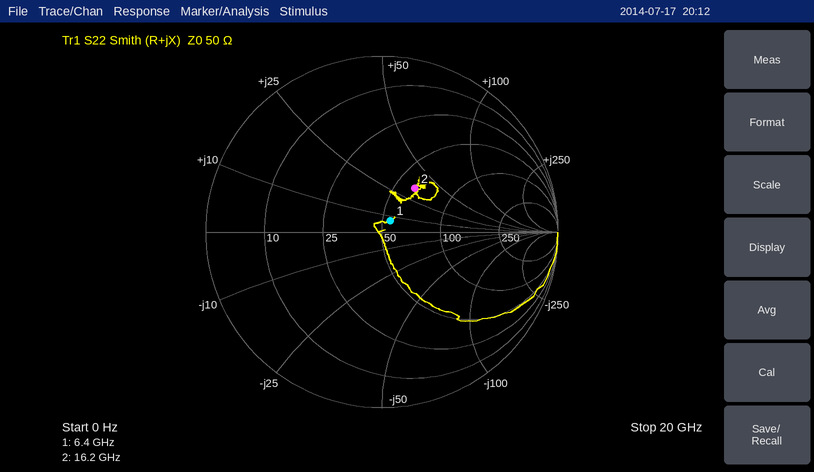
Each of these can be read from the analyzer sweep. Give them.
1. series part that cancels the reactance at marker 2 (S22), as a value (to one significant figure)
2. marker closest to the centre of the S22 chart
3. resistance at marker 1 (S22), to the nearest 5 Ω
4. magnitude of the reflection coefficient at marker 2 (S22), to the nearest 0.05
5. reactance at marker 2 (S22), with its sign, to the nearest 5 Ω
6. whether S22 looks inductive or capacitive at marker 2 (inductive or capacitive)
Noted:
300 fF
marker 1
55 Ω
0.30
+35 Ω
inductive
